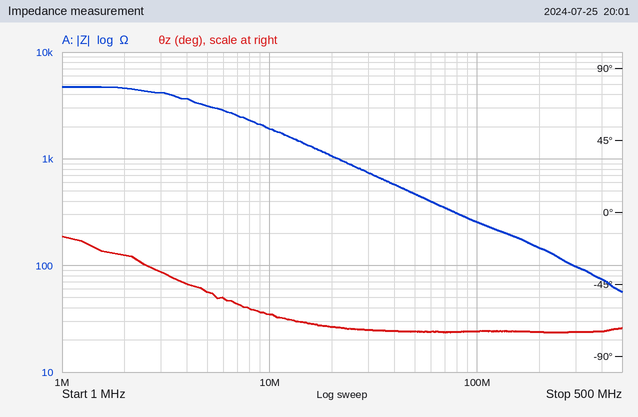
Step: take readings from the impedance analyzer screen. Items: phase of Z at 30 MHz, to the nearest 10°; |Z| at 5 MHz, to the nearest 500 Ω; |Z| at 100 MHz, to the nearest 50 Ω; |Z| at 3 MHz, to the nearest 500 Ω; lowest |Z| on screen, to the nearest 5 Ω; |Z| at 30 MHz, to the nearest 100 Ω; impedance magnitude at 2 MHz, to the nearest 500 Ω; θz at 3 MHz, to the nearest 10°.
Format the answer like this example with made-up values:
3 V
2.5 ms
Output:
-70°
3.0 kΩ
250 Ω
4.0 kΩ
55 Ω
700 Ω
4.5 kΩ
-40°
